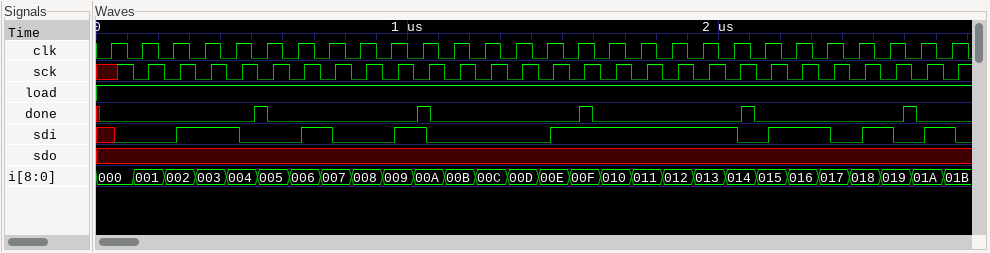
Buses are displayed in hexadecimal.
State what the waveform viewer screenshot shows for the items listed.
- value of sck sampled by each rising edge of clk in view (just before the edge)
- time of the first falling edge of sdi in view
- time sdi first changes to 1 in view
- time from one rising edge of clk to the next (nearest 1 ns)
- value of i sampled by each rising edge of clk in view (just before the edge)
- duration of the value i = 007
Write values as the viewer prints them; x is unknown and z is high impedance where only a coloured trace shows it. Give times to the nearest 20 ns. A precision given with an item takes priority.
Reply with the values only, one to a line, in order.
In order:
x 0 0 0 0 0 0 0 0 0 0 0 0 0 0 0 0 0 0 0 0 0 0 0 0 0 0 0
460 ns
260 ns
100 ns
000, 001, 002, 003, 004, 005, 006, 007, 008, 009, 00A, 00B, 00C, 00D, 00E, 00F, 010, 011, 012, 013, 014, 015, 016, 017, 018, 019, 01A, 01B
100 ns
